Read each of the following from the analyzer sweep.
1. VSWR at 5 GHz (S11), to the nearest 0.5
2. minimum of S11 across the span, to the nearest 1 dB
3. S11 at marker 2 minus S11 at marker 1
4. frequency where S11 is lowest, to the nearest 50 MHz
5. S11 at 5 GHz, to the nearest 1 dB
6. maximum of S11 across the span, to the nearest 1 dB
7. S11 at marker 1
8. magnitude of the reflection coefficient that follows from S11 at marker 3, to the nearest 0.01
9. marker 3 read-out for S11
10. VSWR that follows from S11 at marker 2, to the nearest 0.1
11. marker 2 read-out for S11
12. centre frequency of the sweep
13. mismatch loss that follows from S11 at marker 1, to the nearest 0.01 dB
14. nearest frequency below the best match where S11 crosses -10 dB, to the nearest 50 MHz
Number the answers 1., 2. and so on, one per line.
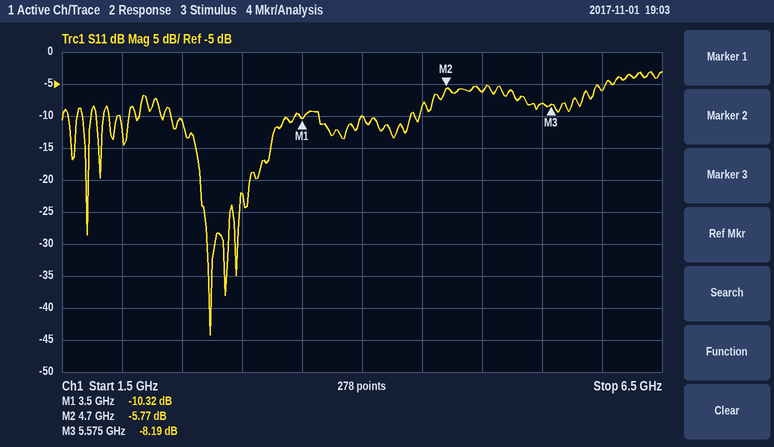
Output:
1. 3.0
2. -44 dB
3. 4.55 dB
4. 2.75 GHz
5. -6 dB
6. -3 dB
7. -10.32 dB
8. 0.39
9. -8.19 dB
10. 3.1
11. -5.77 dB
12. 4 GHz
13. 0.42 dB
14. 2.40 GHz
